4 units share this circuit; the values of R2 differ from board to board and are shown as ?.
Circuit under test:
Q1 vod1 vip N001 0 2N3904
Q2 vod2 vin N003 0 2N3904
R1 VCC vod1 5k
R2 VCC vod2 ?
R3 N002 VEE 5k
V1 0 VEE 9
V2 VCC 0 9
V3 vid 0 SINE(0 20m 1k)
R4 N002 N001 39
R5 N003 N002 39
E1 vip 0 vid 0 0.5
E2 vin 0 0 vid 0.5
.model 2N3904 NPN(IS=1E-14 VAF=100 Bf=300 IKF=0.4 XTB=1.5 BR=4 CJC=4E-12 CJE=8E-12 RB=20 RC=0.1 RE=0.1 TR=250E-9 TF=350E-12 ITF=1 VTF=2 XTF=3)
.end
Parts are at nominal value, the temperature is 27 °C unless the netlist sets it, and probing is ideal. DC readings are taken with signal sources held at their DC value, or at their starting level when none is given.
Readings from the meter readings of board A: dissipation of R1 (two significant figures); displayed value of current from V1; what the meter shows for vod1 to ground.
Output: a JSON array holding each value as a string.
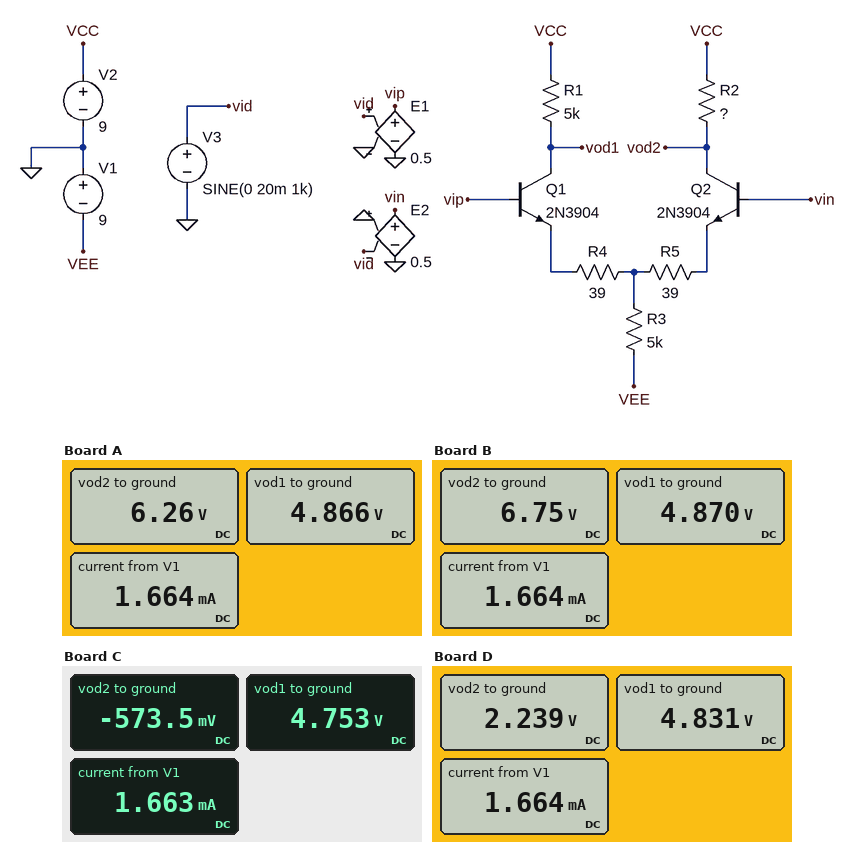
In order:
["3.4 mW", "1.664 mA", "4.866 V"]
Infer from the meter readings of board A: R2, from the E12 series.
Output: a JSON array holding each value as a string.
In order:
["3.3 kΩ"]
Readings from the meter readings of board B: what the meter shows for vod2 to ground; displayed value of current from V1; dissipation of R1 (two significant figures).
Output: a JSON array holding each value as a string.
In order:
["6.75 V", "1.664 mA", "3.4 mW"]
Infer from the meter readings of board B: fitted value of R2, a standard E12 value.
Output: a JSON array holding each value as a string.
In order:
["2.7 kΩ"]
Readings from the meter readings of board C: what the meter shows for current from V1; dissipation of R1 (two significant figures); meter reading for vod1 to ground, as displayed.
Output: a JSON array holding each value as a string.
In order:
["1.663 mA", "3.6 mW", "4.753 V"]
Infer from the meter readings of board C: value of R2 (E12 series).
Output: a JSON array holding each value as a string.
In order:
["12 kΩ"]
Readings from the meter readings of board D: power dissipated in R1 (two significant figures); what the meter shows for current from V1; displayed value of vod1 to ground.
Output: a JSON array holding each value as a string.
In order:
["3.5 mW", "1.664 mA", "4.831 V"]
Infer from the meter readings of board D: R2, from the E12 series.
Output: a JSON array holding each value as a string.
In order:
["8.2 kΩ"]
